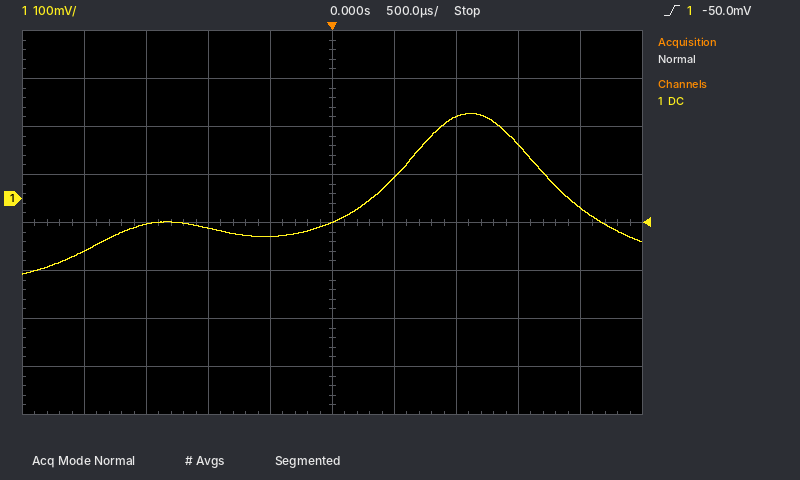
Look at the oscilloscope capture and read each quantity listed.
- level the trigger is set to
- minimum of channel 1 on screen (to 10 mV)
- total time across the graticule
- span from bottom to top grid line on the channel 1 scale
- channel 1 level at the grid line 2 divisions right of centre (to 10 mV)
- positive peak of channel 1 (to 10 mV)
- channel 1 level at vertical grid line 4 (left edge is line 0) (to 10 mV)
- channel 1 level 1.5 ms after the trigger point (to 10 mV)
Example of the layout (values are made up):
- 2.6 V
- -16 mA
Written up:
- -50.0 mV
- -160 mV
- 5 ms
- 800 mV
- 170 mV
- 180 mV
- -80 mV
- 110 mV
